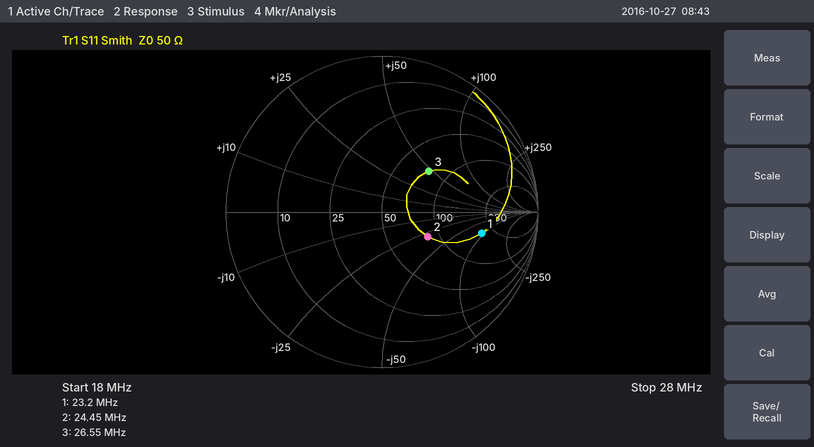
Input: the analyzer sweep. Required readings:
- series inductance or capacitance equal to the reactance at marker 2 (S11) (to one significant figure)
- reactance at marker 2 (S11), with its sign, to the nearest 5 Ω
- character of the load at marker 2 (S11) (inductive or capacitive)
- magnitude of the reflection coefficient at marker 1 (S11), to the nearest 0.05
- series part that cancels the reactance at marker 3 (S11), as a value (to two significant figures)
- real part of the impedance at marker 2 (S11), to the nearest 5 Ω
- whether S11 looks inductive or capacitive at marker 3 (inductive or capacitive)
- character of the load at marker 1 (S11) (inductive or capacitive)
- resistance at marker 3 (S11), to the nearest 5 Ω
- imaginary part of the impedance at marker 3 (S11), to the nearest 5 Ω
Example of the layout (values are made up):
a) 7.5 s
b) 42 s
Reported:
a) 200 pF
b) -30 Ω
c) capacitive
d) 0.65
e) 130 pF
f) 85 Ω
g) inductive
h) capacitive
i) 75 Ω
j) +45 Ω
